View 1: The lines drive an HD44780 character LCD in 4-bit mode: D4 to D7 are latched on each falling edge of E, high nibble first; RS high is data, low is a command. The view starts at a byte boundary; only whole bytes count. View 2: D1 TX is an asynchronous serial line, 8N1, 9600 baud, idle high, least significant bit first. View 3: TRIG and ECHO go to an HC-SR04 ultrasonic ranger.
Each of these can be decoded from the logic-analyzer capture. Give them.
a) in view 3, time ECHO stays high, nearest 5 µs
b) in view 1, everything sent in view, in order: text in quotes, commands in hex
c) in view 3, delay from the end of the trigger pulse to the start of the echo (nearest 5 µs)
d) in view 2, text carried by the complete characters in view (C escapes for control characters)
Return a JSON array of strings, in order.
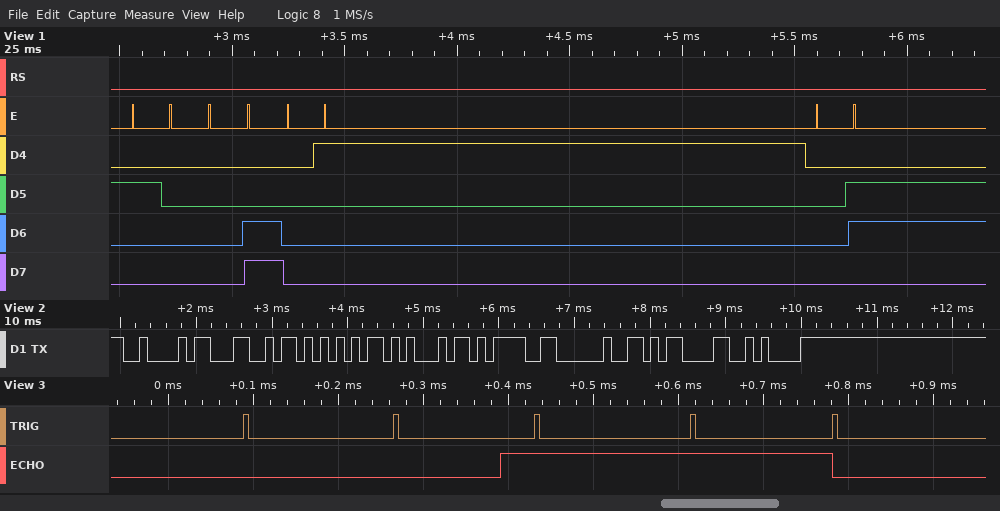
["390 µs", "0x20 0x0C 0x01 0x06", "120 µs", "\"BLUE= \\r\\n\""]
